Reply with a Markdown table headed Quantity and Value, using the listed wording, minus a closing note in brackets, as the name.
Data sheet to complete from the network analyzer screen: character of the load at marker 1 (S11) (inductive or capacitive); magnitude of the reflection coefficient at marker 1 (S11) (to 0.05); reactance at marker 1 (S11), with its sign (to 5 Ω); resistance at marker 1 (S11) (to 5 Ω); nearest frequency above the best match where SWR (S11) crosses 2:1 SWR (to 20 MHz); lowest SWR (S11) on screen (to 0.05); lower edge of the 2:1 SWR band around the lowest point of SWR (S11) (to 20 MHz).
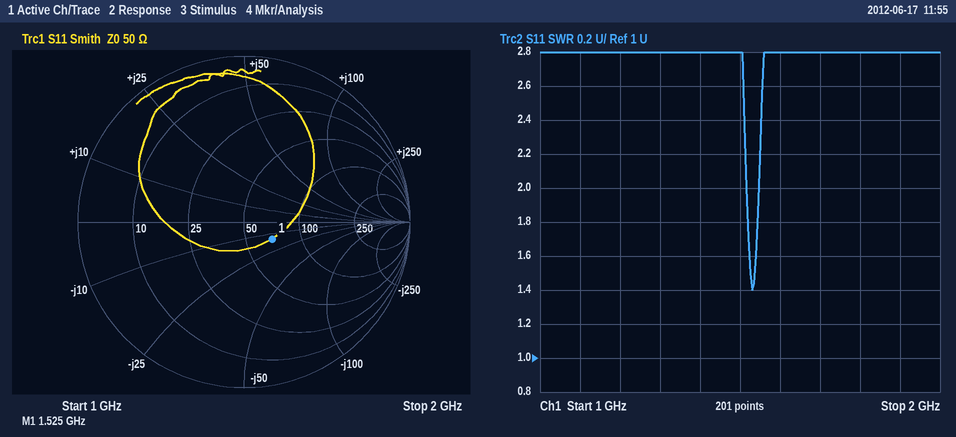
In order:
| Quantity | Value |
|---|---|
| character of the load at marker 1 (S11) | capacitive |
| magnitude of the reflection coefficient at marker 1 (S11) | 0.20 |
| reactance at marker 1 (S11), with its sign | -15 Ω |
| resistance at marker 1 (S11) | 70 Ω |
| nearest frequency above the best match where SWR (S11) crosses 2:1 SWR | 1.54 GHz |
| lowest SWR (S11) on screen | 1.40 |
| lower edge of the 2:1 SWR band around the lowest point of SWR (S11) | 1.52 GHz |
